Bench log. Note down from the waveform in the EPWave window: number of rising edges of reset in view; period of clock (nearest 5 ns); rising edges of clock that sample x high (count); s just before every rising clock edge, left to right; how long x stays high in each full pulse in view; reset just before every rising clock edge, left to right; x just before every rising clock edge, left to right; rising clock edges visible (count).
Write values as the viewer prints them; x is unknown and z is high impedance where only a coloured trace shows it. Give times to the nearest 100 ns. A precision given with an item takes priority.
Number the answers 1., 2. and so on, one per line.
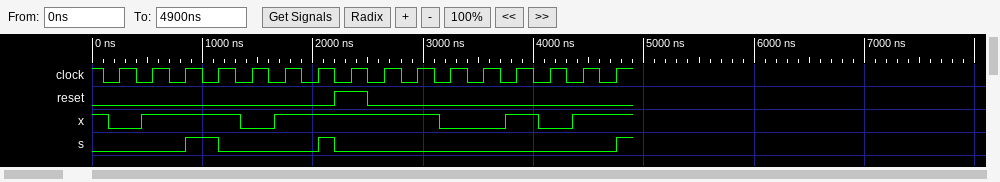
1. 1
2. 300 ns
3. 11
4. 0 0 0 1 0 0 0 0 0 0 0 0 0 0 0 0
5. 900 ns, 1500 ns, 300 ns
6. 0 0 0 0 0 0 0 1 0 0 0 0 0 0 0 0
7. 0 1 1 1 0 1 1 1 1 1 0 0 1 0 1 1
8. 16
